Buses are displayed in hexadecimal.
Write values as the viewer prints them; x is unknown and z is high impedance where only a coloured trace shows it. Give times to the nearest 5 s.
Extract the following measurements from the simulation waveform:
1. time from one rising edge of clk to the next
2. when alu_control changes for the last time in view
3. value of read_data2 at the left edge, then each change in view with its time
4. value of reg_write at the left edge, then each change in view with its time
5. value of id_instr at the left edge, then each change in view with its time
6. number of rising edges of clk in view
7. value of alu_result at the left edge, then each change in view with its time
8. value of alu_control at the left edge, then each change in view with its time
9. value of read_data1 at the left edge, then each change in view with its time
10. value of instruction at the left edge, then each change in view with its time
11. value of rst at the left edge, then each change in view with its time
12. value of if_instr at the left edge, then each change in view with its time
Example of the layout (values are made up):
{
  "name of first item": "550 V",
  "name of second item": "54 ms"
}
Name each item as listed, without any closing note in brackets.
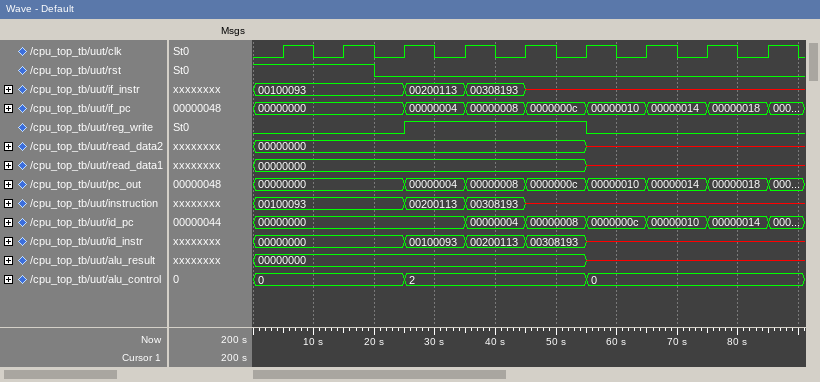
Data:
{
  "time from one rising edge of clk to the next": "10 s",
  "when alu_control changes for the last time in view": "55 s",
  "value of read_data2 at the left edge, then each change in view with its time": "00000000, x at 55 s",
  "value of reg_write at the left edge, then each change in view with its time": "0, 1 at 25 s, 0 at 55 s",
  "value of id_instr at the left edge, then each change in view with its time": "00000000, 00100093 at 25 s, 00200113 at 35 s, 00308193 at 45 s, x at 55 s",
  "number of rising edges of clk in view": "9",
  "value of alu_result at the left edge, then each change in view with its time": "00000000, x at 55 s",
  "value of alu_control at the left edge, then each change in view with its time": "0, 2 at 25 s, 0 at 55 s",
  "value of read_data1 at the left edge, then each change in view with its time": "00000000, x at 55 s",
  "value of instruction at the left edge, then each change in view with its time": "00100093, 00200113 at 25 s, 00308193 at 35 s, x at 45 s",
  "value of rst at the left edge, then each change in view with its time": "1, 0 at 20 s",
  "value of if_instr at the left edge, then each change in view with its time": "00100093, 00200113 at 25 s, 00308193 at 35 s, x at 45 s"
}
